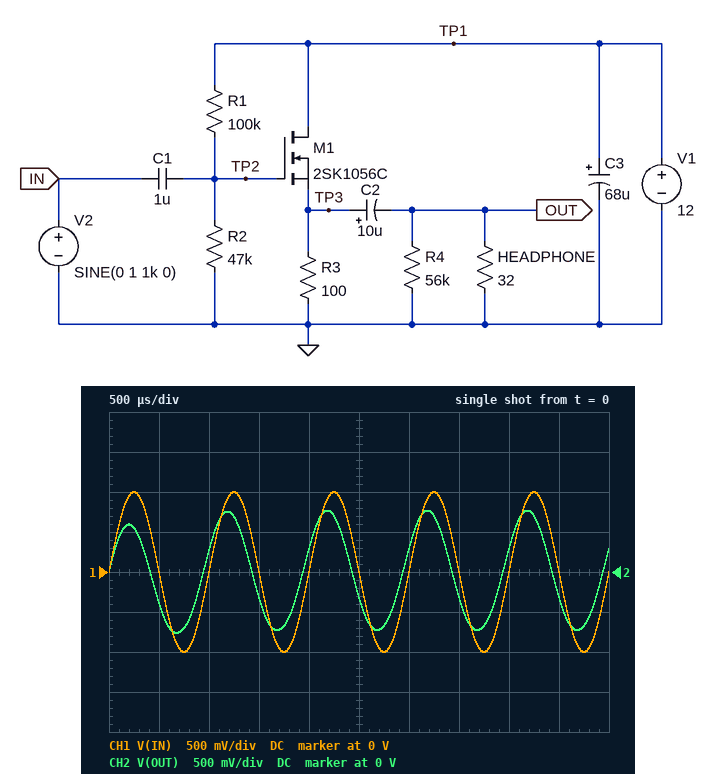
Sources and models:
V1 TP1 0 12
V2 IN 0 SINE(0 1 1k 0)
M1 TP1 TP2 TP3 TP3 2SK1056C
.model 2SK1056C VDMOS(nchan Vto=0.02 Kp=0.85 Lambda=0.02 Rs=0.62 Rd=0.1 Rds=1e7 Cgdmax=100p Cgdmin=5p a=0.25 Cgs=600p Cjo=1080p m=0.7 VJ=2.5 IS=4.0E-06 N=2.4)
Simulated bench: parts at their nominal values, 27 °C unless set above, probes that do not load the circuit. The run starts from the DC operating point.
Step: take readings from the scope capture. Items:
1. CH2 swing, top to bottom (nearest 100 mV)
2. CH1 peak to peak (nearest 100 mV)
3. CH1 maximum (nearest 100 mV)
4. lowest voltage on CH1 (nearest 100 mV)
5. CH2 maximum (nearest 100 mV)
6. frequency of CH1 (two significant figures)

1.5 V
2.0 V
1.0 V
-1.0 V
800 mV
1.0 kHz
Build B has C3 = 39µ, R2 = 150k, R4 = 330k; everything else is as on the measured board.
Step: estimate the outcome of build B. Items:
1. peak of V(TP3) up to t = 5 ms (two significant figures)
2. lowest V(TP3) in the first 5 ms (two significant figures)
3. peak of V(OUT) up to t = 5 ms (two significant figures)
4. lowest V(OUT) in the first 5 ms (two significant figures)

7.7 V
5.9 V
800 mV
-830 mV
